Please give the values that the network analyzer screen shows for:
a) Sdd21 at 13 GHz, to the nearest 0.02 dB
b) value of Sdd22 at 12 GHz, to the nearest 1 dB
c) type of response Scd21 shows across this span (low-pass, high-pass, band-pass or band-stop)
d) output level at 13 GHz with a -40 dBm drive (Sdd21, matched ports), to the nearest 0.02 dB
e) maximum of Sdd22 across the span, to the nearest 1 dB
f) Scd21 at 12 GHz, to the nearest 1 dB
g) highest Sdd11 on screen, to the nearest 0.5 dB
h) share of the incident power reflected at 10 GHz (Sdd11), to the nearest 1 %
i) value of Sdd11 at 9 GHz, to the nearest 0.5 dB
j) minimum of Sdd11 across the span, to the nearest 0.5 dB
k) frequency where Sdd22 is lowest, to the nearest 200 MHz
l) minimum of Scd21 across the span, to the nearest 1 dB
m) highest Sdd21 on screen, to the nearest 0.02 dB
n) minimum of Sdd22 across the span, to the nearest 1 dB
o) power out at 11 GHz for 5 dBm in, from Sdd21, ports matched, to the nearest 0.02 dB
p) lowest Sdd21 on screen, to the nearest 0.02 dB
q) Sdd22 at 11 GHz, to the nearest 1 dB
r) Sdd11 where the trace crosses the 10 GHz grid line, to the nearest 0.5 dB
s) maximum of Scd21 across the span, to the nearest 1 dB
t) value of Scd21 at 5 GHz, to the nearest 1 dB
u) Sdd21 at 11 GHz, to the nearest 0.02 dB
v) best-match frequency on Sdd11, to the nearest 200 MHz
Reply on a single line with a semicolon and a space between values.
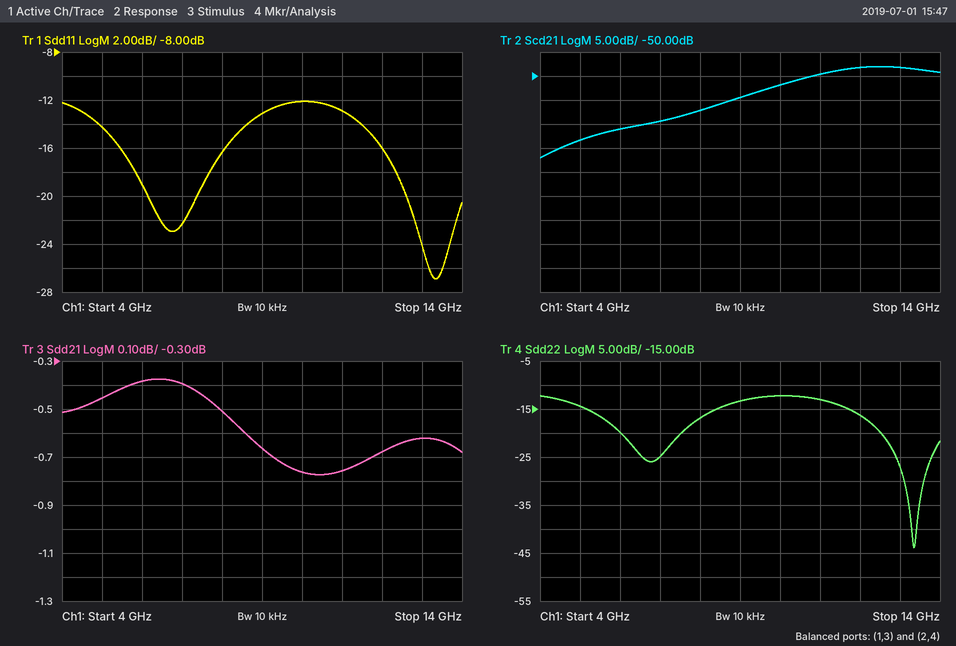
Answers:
-0.62 dB; -16 dB; high-pass; -40.62 dBm; -12 dB; -48 dB; -12.0 dB; 6 %; -13.0 dB; -27.0 dB; 13.4 GHz; -67 dB; -0.38 dB; -44 dB; 4.24 dBm; -0.78 dB; -13 dB; -12.0 dB; -48 dB; -63 dB; -0.76 dB; 13.4 GHz
